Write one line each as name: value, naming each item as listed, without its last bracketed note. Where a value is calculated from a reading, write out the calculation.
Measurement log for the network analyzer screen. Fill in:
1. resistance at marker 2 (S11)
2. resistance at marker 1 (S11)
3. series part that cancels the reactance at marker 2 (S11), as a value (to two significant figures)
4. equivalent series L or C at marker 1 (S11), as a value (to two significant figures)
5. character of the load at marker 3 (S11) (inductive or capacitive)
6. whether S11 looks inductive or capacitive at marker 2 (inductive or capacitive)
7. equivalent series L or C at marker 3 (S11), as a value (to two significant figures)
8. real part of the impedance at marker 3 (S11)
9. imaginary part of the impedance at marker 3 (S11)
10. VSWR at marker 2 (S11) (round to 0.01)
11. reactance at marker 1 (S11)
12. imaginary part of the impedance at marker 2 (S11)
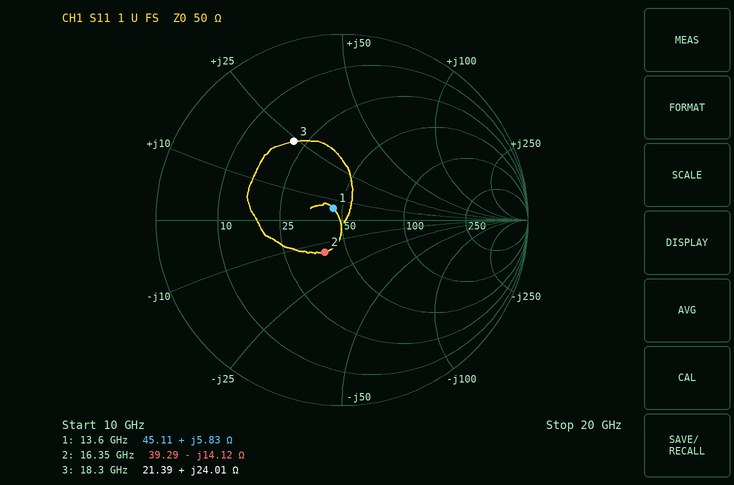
resistance at marker 2: 39.29 Ω
resistance at marker 1: 45.11 Ω
series part that cancels the reactance at marker 2 (S11), as a value: L = 14.12 Ω/(2π × 16.35 GHz) ≈ 137 pH, so 140 pH to two significant figures
equivalent series L or C at marker 1 (S11), as a value: L = 5.83 Ω/(2π × 13.6 GHz) ≈ 68 pH
character of the load at marker 3 (S11): inductive
whether S11 looks inductive or capacitive at marker 2: capacitive
equivalent series L or C at marker 3 (S11), as a value: L = 24.01 Ω/(2π × 18.3 GHz) ≈ 209 pH, so 210 pH to two significant figures
real part of the impedance at marker 3: 21.39 Ω
imaginary part of the impedance at marker 3: +24.01 Ω
VSWR at marker 2 (S11): 1.49
reactance at marker 1: +5.83 Ω
imaginary part of the impedance at marker 2: -14.12 Ω
